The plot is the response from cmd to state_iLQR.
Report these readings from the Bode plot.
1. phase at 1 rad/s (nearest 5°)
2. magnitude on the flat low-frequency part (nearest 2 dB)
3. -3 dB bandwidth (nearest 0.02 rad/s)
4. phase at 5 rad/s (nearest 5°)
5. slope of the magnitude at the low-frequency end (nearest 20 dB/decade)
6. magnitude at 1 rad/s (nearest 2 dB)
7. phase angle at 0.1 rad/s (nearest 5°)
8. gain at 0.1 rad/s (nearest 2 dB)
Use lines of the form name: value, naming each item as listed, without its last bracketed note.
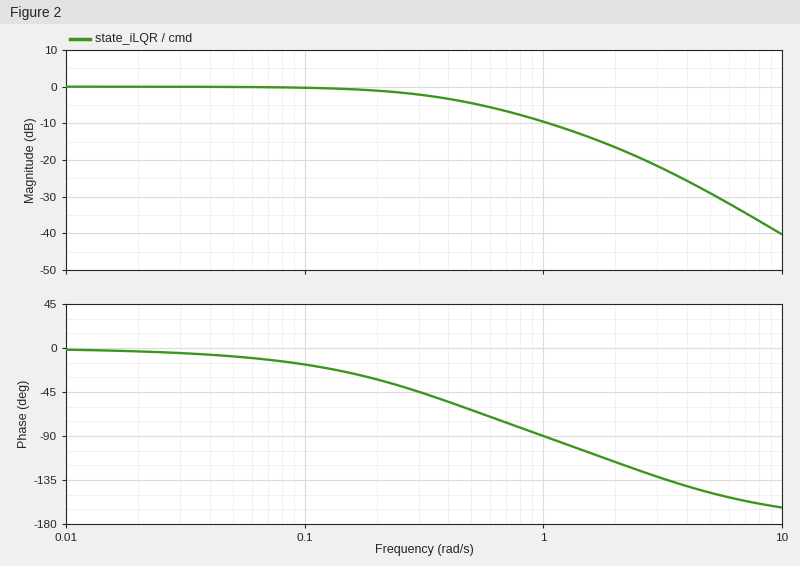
phase at 1 rad/s: -90°
magnitude on the flat low-frequency part: 0 dB
-3 dB bandwidth: 0.38 rad/s
phase at 5 rad/s: -150°
slope of the magnitude at the low-frequency end: 0 dB/decade
magnitude at 1 rad/s: -10 dB
phase angle at 0.1 rad/s: -15°
gain at 0.1 rad/s: 0 dB
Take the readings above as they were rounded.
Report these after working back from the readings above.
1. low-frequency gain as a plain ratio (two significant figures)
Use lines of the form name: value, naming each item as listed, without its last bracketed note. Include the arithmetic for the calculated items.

low-frequency gain as a plain ratio: 10^(0 / 20) = 1.0
